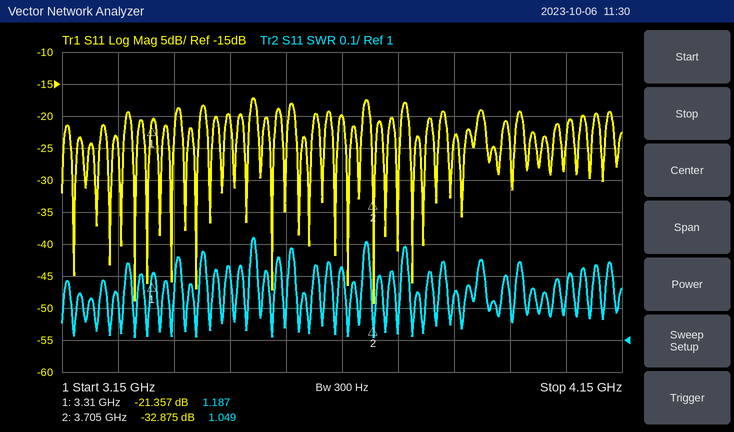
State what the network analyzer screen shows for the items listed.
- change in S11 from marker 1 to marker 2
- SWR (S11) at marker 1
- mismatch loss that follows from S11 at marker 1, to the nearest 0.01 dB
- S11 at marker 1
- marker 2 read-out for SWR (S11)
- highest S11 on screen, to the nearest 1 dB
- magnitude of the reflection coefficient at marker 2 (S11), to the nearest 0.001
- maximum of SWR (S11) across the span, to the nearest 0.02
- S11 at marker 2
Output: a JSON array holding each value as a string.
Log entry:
["-11.518 dB", "1.187", "0.03 dB", "-21.357 dB", "1.049", "-17 dB", "0.023", "1.32", "-32.875 dB"]
